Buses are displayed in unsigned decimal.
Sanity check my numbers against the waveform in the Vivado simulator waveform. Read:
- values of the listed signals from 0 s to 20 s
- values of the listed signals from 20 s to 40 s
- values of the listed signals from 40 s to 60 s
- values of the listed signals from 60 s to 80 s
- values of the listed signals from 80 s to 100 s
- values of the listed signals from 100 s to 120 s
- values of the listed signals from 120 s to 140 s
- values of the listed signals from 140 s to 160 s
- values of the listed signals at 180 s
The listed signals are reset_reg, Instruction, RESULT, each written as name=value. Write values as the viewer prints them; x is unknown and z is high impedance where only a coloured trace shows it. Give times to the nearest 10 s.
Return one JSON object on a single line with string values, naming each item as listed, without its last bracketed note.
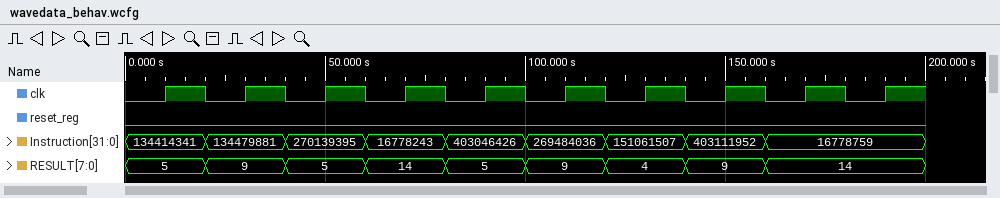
{"values of the listed signals from 0 s to 20 s": "reset_reg=0, Instruction=134414341, RESULT=5", "values of the listed signals from 20 s to 40 s": "reset_reg=0, Instruction=134479881, RESULT=9", "values of the listed signals from 40 s to 60 s": "reset_reg=0, Instruction=270139395, RESULT=5", "values of the listed signals from 60 s to 80 s": "reset_reg=0, Instruction=16778243, RESULT=14", "values of the listed signals from 80 s to 100 s": "reset_reg=0, Instruction=403046426, RESULT=5", "values of the listed signals from 100 s to 120 s": "reset_reg=0, Instruction=269484036, RESULT=9", "values of the listed signals from 120 s to 140 s": "reset_reg=0, Instruction=151061507, RESULT=4", "values of the listed signals from 140 s to 160 s": "reset_reg=0, Instruction=403111952, RESULT=9", "values of the listed signals at 180 s": "reset_reg=0, Instruction=16778759, RESULT=14"}
